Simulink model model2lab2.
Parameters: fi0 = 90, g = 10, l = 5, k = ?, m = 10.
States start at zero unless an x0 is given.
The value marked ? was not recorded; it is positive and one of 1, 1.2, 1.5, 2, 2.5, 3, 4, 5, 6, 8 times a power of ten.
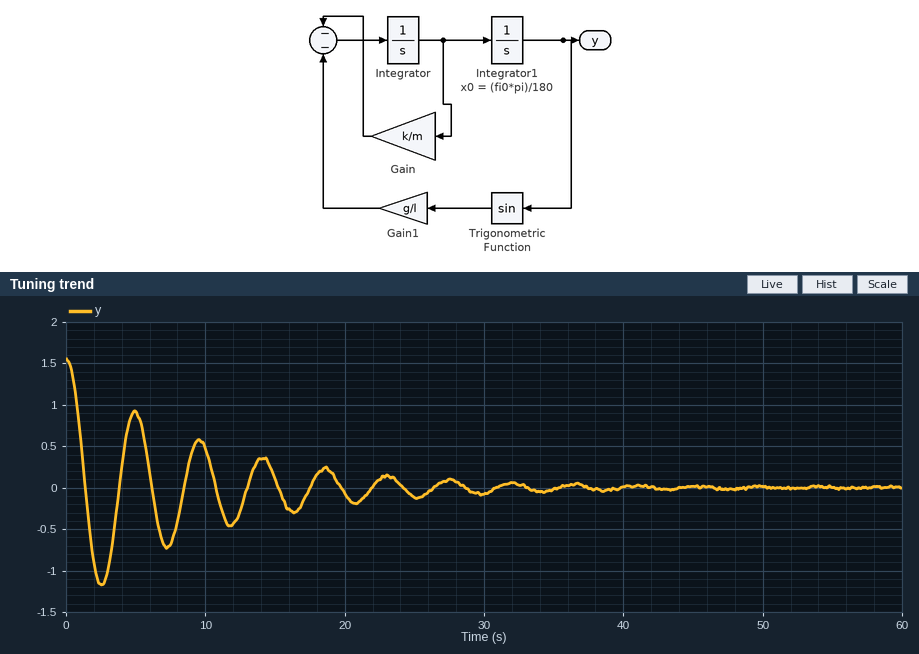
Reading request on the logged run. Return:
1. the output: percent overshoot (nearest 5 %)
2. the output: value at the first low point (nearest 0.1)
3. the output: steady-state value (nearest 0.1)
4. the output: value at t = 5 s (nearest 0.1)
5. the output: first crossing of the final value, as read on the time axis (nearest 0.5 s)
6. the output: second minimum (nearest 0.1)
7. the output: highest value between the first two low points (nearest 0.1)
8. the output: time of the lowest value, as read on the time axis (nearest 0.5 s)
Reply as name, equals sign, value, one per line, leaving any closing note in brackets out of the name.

the output: percent overshoot = 75 %
the output: value at the first low point = -1.2
the output: steady-state value = 0.0
the output: value at t = 5 s = 0.9
the output: first crossing of the final value, as read on the time axis = 1.5 s
the output: second minimum = -0.7
the output: highest value between the first two low points = 0.9
the output: time of the lowest value, as read on the time axis = 2.5 s
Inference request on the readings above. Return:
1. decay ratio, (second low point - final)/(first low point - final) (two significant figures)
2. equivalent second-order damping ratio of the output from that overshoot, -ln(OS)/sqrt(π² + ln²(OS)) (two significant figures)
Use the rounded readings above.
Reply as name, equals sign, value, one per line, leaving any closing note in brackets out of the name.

decay ratio, (second low point - final)/(first low point - final) = 0.58
equivalent second-order damping ratio of the output from that overshoot, -ln(OS)/sqrt(π² + ln²(OS)) = 0.091
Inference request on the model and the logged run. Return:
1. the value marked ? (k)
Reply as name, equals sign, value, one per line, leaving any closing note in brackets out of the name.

the value marked ? = 2
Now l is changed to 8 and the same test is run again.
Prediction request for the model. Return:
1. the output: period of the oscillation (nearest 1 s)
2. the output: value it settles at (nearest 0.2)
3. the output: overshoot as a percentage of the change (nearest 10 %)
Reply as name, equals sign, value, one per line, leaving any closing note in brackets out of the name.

the output: period of the oscillation = 6 s
the output: value it settles at = 0.0
the output: overshoot as a percentage of the change = 70 %
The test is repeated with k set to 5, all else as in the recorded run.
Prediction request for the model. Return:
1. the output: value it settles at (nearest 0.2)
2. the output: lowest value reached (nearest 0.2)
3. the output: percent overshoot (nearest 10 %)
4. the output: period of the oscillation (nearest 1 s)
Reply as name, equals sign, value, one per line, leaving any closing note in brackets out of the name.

the output: value it settles at = 0.0
the output: lowest value reached = -0.8
the output: percent overshoot = 50 %
the output: period of the oscillation = 5 s
